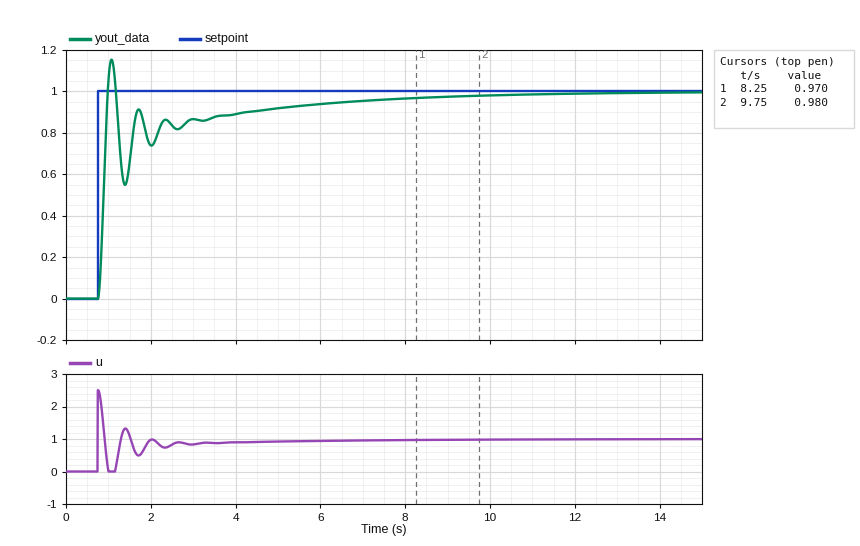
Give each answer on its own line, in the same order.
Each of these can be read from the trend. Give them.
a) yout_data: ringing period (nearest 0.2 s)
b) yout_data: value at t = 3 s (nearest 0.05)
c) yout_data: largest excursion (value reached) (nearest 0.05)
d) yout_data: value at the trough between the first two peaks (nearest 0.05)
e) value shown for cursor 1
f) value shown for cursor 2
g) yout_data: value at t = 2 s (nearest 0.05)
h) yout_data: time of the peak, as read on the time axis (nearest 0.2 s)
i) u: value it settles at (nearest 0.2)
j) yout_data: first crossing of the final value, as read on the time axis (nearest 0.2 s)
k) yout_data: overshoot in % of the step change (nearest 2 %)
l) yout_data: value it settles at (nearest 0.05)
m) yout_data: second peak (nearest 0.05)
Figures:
0.6 s
0.85
1.15
0.55
0.970
0.980
0.75
1.0 s
1.0
1.0 s
16 %
1.00
0.90
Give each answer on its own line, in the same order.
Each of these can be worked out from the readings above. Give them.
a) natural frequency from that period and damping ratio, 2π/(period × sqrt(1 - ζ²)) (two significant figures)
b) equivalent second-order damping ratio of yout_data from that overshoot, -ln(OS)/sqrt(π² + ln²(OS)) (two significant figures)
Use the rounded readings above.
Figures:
12 rad/s
0.50
